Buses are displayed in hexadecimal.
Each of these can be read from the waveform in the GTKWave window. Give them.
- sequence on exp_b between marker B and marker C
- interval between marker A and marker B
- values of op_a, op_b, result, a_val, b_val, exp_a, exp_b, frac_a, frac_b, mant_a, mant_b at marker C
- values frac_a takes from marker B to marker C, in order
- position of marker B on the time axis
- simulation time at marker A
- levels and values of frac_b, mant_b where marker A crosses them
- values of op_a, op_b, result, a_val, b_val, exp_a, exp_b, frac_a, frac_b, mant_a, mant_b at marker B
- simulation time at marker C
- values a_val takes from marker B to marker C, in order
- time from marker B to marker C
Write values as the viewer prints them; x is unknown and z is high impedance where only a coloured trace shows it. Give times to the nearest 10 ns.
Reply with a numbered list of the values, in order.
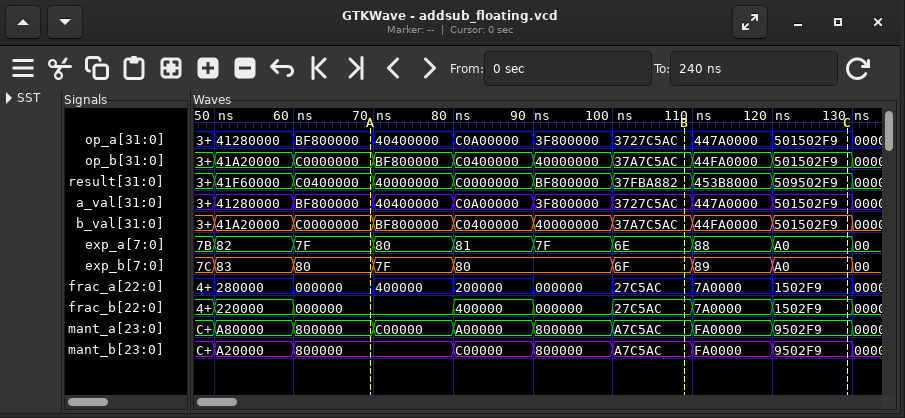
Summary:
1. 6F, 89, A0
2. 40 ns
3. op_a=501502F9, op_b=501502F9, result=509502F9, a_val=501502F9, b_val=501502F9, exp_a=A0, exp_b=A0, frac_a=1502F9, frac_b=1502F9, mant_a=9502F9, mant_b=9502F9
4. 27C5AC, 7A0000, 1502F9
5. 110 ns
6. 70 ns
7. frac_b=000000, mant_b=800000
8. op_a=3727C5AC, op_b=37A7C5AC, result=37FBA882, a_val=3727C5AC, b_val=37A7C5AC, exp_a=6E, exp_b=6F, frac_a=27C5AC, frac_b=27C5AC, mant_a=A7C5AC, mant_b=A7C5AC
9. 130 ns
10. 3727C5AC, 447A0000, 501502F9
11. 20 ns
